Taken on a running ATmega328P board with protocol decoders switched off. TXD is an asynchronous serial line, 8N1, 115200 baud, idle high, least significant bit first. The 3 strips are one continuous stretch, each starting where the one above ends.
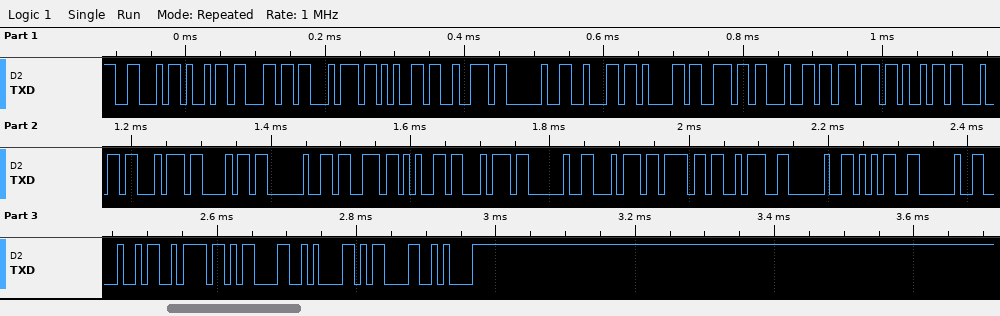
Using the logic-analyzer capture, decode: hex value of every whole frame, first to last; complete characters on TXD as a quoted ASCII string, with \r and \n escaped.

46 69 6C 74 65 72 20 62 61 6E 64 77 69 64 74 68 20 73 65 74 20 74 6F 3A 20 35 20 48 7A 0D 0A 0D 0A
"Filter bandwidth set to: 5 Hz\r\n\r\n"
